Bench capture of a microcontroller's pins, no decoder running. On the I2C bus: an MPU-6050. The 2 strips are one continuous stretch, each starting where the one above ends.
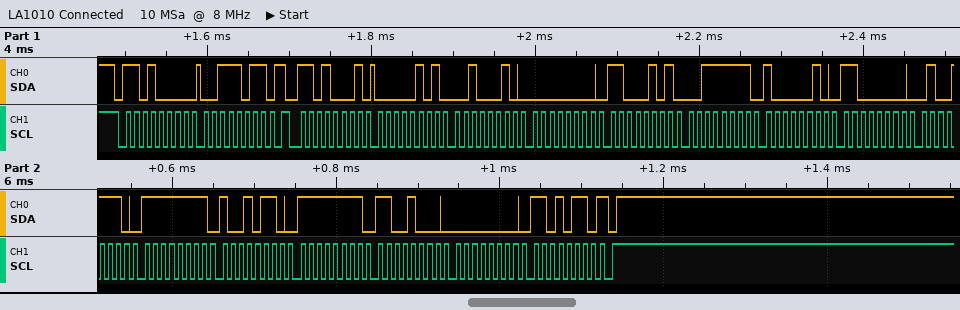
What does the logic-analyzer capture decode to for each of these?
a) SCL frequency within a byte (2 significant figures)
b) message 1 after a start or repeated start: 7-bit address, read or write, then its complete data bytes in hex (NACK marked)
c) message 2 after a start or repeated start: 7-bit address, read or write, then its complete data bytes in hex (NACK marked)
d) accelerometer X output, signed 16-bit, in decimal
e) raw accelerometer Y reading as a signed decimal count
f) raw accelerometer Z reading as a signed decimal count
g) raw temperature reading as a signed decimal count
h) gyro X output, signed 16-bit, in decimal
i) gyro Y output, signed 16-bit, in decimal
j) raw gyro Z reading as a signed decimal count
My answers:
100 kHz
0x68 write: 3B
0x68 read: 05 22 00 C5 3F 82 C0 4E FF 96 FF C8 00 D6 NACK
1314
197
16258
-16306
-106
-56
214
